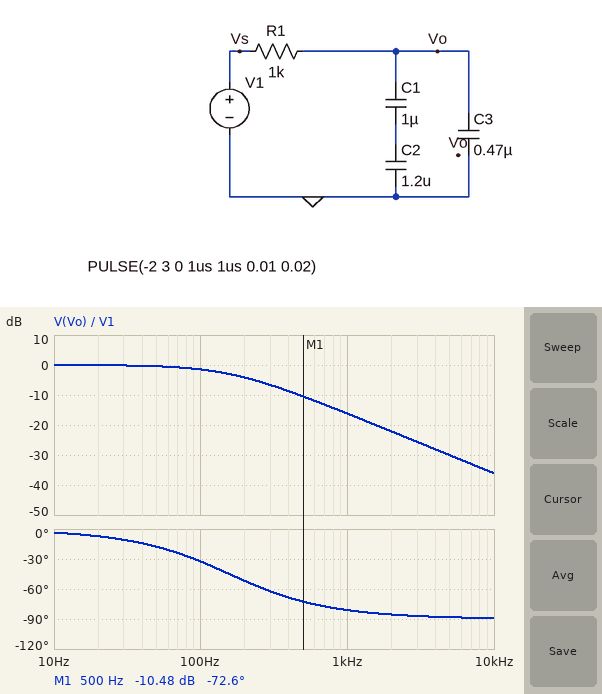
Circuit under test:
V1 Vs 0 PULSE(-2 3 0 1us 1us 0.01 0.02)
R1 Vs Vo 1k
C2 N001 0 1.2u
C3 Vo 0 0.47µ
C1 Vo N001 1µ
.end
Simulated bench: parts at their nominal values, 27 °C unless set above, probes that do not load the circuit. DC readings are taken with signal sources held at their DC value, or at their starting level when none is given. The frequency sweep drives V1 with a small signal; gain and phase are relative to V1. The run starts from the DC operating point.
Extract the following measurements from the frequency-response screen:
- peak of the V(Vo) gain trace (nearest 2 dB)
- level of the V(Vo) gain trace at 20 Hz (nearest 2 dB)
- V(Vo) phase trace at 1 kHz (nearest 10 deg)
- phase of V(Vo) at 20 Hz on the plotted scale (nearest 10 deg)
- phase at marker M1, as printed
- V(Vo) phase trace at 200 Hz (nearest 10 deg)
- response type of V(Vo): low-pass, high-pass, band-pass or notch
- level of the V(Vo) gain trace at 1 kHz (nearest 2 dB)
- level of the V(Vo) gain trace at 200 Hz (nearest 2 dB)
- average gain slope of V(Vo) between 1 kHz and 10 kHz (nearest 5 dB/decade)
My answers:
0 dB
0 dB
-80 deg
-10 deg
-72.6 deg
-50 deg
low-pass
-16 dB
-4 dB
-20 dB/decade
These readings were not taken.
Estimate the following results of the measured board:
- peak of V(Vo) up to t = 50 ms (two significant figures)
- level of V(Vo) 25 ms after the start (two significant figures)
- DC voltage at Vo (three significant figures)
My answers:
3.0 V
3.0 V
-2.00 V
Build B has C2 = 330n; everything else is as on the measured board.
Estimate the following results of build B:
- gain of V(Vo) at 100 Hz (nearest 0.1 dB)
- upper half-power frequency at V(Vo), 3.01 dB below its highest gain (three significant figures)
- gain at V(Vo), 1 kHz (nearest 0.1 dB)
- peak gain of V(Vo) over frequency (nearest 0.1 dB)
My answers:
-0.8 dB
222 Hz
-13.3 dB
0 dB
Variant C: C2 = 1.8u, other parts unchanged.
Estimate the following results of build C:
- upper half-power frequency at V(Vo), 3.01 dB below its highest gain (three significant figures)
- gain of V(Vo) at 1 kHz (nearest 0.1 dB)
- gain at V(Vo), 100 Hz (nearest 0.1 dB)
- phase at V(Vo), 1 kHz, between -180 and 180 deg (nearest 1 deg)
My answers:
143 Hz
-17.0 dB
-1.7 dB
-82 deg
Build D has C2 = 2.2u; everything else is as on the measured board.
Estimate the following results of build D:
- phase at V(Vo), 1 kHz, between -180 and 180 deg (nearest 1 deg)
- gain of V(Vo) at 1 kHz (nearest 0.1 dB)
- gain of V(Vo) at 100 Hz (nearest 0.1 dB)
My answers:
-82 deg
-17.3 dB
-1.8 dB
